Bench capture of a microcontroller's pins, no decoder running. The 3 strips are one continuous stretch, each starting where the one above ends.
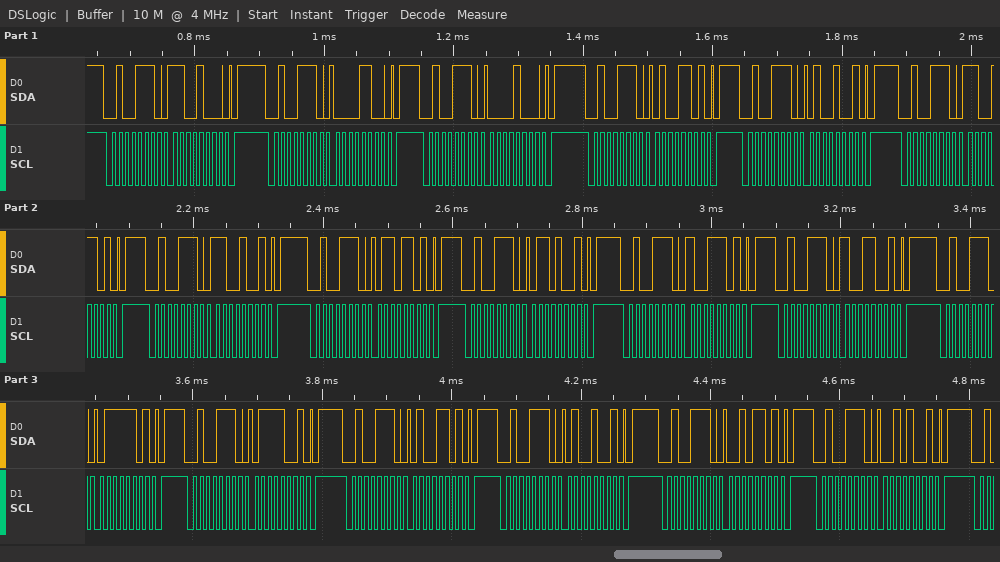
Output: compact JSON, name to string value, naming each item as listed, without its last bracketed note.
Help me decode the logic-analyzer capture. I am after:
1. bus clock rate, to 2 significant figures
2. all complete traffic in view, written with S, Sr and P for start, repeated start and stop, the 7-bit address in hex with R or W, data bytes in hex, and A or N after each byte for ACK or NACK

{"bus clock rate, to 2 significant figures": "100 kHz", "all complete traffic in view, written with S, Sr and P for start, repeated start and stop, the 7-bit address in hex with R or W, data bytes in hex, and A or N after each byte for ACK or NACK": "S 27W A C8 A P S 27W A 0C A P S 27W A 08 A P S 27W A 4D A P S 27W A 49 A P S 27W A CD A P S 27W A C9 A P S 27W A 6D A P S 27W A 69 A P S 27W A 9D A P S 27W A 99 A P S 27W A 7D A P S 27W A 79 A P S 27W A 4D A P S 27W A 49 A P S 27W A 2D A P S 27W A 29 A P"}
